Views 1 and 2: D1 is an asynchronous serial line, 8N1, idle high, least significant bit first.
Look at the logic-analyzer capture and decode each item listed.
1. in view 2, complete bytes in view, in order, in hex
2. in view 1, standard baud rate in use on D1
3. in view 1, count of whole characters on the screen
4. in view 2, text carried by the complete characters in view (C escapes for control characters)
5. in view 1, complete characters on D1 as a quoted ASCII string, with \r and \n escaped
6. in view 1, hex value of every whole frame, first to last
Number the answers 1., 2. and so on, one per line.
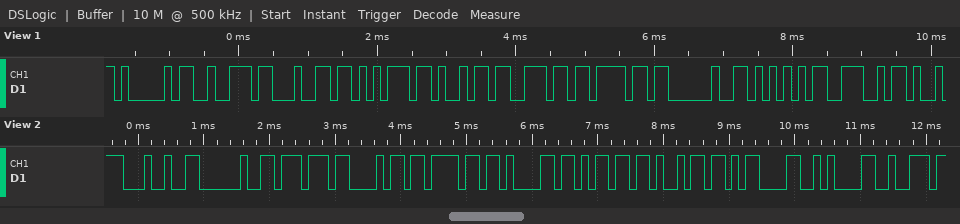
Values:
1. 0x24 0x20 0x77 0x68 0x6F 0x61 0x6D 0x69 0x0D 0x0A 0x72
2. 9600 baud
3. 10
4. "$ whoami\r\nr"
5. "Arduino UN"
6. 41 72 64 75 69 6E 6F 20 55 4E
